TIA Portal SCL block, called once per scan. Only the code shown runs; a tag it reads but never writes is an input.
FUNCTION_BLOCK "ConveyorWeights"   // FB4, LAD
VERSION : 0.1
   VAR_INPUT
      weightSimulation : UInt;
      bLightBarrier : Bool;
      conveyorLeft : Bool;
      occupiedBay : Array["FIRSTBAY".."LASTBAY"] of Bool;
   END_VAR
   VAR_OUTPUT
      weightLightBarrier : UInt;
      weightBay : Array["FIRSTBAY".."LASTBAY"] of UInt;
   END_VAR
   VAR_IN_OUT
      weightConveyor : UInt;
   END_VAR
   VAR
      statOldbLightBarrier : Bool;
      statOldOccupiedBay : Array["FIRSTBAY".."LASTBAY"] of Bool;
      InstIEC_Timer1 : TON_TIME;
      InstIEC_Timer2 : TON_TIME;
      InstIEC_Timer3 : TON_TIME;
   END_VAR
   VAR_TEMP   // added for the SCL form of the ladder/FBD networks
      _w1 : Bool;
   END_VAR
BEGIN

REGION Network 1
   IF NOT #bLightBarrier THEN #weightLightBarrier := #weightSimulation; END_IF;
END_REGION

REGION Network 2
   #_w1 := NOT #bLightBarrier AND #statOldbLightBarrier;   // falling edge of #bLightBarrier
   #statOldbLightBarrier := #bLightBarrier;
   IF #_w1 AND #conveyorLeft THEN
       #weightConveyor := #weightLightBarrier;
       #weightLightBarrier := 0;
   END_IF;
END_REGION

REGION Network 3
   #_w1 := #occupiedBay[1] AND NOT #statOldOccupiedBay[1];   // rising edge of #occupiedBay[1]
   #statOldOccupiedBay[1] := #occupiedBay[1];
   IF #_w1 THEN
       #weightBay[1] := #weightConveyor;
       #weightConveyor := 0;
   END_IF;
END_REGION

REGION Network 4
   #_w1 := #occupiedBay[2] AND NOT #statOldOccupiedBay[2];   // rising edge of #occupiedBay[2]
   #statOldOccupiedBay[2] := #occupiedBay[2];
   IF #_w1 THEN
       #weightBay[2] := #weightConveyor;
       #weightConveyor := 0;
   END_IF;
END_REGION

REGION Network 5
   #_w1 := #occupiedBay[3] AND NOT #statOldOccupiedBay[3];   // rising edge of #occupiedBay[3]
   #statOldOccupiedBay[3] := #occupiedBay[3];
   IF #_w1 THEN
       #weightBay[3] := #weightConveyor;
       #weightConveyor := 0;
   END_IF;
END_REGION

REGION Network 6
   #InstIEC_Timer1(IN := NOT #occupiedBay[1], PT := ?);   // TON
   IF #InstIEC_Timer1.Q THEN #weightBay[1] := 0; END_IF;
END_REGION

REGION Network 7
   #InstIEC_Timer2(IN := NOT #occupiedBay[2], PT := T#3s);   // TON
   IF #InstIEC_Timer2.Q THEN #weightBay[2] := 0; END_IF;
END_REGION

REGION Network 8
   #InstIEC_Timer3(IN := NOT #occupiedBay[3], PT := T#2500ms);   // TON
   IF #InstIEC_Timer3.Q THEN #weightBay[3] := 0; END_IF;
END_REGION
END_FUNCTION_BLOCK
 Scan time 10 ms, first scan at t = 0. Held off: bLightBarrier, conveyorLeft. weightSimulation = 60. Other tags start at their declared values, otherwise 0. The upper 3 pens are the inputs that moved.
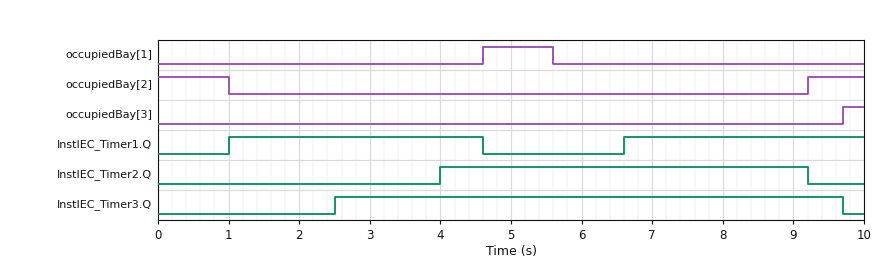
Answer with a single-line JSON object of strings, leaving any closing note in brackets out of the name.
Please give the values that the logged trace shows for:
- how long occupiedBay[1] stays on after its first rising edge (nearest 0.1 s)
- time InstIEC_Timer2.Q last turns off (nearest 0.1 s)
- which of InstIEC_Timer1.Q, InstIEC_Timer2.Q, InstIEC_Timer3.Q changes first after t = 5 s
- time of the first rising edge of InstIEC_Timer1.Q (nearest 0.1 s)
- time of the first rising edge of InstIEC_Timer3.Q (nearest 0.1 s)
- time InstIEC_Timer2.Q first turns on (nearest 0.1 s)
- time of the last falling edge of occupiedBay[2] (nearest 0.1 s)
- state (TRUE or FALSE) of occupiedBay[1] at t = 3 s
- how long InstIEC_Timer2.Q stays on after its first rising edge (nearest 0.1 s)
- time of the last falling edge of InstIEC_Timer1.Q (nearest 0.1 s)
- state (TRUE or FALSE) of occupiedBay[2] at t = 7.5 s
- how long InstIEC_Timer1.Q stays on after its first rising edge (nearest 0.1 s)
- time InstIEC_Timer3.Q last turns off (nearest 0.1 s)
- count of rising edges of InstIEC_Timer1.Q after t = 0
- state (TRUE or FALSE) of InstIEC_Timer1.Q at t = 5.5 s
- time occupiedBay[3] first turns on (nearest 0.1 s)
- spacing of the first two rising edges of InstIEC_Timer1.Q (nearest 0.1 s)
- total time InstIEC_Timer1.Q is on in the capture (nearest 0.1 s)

{"how long occupiedBay[1] stays on after its first rising edge": "1.0 s", "time InstIEC_Timer2.Q last turns off": "9.2 s", "which of InstIEC_Timer1.Q, InstIEC_Timer2.Q, InstIEC_Timer3.Q changes first after t = 5 s": "InstIEC_Timer1.Q", "time of the first rising edge of InstIEC_Timer1.Q": "1.0 s", "time of the first rising edge of InstIEC_Timer3.Q": "2.5 s", "time InstIEC_Timer2.Q first turns on": "4.0 s", "time of the last falling edge of occupiedBay[2]": "1.0 s", "state (TRUE or FALSE) of occupiedBay[1] at t = 3 s": "FALSE", "how long InstIEC_Timer2.Q stays on after its first rising edge": "5.2 s", "time of the last falling edge of InstIEC_Timer1.Q": "4.6 s", "state (TRUE or FALSE) of occupiedBay[2] at t = 7.5 s": "FALSE", "how long InstIEC_Timer1.Q stays on after its first rising edge": "3.6 s", "time InstIEC_Timer3.Q last turns off": "9.7 s", "count of rising edges of InstIEC_Timer1.Q after t = 0": "2", "state (TRUE or FALSE) of InstIEC_Timer1.Q at t = 5.5 s": "FALSE", "time occupiedBay[3] first turns on": "9.7 s", "spacing of the first two rising edges of InstIEC_Timer1.Q": "5.6 s", "total time InstIEC_Timer1.Q is on in the capture": "7.0 s"}
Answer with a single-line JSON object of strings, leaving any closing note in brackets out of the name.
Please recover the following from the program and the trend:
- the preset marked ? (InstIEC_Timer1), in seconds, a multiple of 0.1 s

{"the preset marked ? (InstIEC_Timer1), in seconds, a multiple of 0.1 s": "1.0 s"}
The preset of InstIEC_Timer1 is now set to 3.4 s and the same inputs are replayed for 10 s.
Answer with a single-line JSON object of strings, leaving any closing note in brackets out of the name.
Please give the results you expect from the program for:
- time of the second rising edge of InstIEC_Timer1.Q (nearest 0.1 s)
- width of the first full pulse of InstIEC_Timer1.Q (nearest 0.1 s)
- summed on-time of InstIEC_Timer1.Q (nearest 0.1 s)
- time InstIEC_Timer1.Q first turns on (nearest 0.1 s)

{"time of the second rising edge of InstIEC_Timer1.Q": "9.0 s", "width of the first full pulse of InstIEC_Timer1.Q": "1.2 s", "summed on-time of InstIEC_Timer1.Q": "2.2 s", "time InstIEC_Timer1.Q first turns on": "3.4 s"}
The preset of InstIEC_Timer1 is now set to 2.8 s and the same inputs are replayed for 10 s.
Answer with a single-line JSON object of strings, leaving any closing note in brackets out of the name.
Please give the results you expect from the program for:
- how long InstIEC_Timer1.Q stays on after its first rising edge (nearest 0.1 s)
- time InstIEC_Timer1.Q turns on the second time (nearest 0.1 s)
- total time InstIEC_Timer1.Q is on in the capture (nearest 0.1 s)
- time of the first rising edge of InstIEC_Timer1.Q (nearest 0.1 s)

{"how long InstIEC_Timer1.Q stays on after its first rising edge": "1.8 s", "time InstIEC_Timer1.Q turns on the second time": "8.4 s", "total time InstIEC_Timer1.Q is on in the capture": "3.4 s", "time of the first rising edge of InstIEC_Timer1.Q": "2.8 s"}
